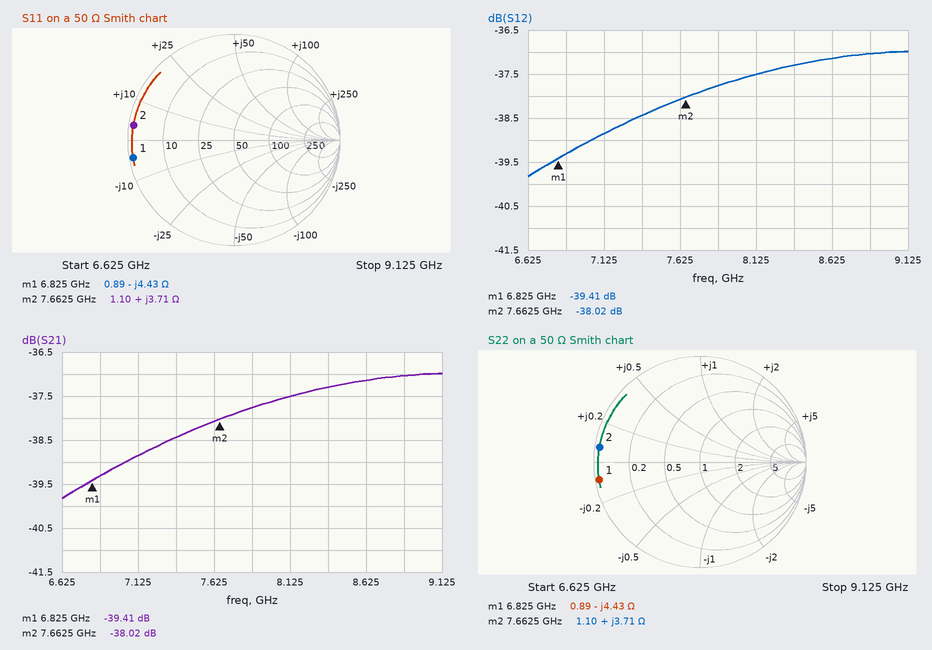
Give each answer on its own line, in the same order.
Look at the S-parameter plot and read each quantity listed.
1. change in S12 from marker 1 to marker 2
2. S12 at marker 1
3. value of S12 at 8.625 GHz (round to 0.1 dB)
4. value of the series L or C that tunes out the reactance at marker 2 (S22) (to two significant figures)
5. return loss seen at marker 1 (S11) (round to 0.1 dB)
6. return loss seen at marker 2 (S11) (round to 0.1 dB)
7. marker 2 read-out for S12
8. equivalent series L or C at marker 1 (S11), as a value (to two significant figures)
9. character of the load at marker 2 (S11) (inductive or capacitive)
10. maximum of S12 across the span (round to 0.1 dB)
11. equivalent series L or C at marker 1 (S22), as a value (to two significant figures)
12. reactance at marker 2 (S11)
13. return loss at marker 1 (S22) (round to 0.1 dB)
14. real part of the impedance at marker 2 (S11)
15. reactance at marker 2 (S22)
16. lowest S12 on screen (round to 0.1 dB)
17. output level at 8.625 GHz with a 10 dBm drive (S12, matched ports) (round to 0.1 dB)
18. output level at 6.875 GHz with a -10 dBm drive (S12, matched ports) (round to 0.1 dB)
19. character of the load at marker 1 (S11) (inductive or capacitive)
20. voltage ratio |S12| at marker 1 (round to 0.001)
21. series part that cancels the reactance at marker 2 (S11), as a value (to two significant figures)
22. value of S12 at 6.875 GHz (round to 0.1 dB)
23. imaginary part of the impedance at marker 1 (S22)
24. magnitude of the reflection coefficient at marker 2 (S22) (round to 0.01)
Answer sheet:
1.39 dB
-39.41 dB
-37.1 dB
5.6 pF
0.3 dB
0.4 dB
-38.02 dB
5.3 pF
inductive
-37.0 dB
5.3 pF
+3.71 Ω
0.3 dB
1.10 Ω
+3.71 Ω
-39.8 dB
-27.1 dBm
-49.3 dBm
capacitive
0.011
5.6 pF
-39.3 dB
-4.43 Ω
0.96
